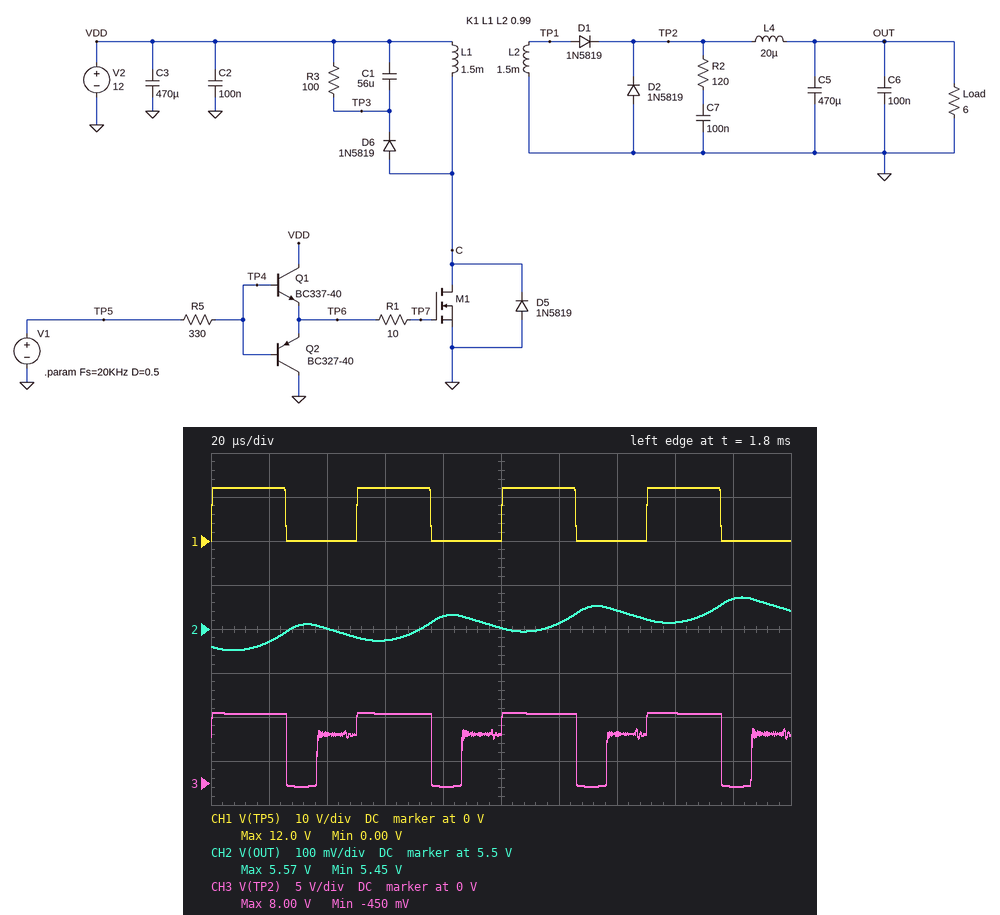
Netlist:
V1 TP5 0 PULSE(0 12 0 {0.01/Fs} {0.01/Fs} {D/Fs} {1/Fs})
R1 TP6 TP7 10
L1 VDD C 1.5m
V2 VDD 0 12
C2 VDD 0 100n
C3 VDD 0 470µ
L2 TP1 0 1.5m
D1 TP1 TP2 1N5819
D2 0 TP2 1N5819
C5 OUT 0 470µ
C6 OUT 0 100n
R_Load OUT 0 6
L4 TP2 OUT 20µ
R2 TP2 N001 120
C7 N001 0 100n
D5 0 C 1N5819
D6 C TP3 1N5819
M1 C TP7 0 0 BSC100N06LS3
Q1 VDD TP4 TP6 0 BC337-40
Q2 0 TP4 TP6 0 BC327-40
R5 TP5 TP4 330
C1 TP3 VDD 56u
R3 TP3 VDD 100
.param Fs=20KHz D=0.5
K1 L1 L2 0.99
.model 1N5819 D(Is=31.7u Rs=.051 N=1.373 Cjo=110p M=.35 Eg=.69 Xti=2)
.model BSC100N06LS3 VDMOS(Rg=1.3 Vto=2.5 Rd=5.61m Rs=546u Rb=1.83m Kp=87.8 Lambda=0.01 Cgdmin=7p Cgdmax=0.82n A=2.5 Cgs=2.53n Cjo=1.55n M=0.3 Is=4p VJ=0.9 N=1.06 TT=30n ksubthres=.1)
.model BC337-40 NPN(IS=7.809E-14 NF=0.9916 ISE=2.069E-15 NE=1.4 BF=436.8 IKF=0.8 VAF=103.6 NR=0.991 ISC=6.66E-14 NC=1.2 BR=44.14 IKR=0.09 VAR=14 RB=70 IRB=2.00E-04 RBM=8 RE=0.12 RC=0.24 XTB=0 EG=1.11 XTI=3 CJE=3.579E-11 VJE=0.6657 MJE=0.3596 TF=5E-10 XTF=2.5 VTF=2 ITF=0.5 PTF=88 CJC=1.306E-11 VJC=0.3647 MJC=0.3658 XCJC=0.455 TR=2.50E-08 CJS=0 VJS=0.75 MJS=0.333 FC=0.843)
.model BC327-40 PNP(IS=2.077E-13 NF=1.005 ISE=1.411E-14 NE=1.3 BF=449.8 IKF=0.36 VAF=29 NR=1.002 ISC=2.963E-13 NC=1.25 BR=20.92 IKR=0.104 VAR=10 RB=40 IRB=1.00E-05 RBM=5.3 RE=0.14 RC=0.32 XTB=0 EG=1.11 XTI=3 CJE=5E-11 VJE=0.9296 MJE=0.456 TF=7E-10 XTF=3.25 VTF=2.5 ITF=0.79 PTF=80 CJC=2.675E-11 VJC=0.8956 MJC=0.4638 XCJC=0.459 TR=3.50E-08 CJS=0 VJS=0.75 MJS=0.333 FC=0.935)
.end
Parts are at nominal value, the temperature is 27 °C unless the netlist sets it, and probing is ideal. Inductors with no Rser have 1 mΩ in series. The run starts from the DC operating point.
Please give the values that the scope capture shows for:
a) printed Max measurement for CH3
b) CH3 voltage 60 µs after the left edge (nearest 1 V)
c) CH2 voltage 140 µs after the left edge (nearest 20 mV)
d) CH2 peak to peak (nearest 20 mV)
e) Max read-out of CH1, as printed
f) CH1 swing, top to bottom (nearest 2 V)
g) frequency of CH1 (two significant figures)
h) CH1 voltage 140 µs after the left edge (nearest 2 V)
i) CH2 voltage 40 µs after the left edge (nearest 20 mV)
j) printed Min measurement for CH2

8.00 V
8 V
5.54 V
120 mV
12.0 V
12 V
20 kHz
0 V
5.50 V
5.45 V
